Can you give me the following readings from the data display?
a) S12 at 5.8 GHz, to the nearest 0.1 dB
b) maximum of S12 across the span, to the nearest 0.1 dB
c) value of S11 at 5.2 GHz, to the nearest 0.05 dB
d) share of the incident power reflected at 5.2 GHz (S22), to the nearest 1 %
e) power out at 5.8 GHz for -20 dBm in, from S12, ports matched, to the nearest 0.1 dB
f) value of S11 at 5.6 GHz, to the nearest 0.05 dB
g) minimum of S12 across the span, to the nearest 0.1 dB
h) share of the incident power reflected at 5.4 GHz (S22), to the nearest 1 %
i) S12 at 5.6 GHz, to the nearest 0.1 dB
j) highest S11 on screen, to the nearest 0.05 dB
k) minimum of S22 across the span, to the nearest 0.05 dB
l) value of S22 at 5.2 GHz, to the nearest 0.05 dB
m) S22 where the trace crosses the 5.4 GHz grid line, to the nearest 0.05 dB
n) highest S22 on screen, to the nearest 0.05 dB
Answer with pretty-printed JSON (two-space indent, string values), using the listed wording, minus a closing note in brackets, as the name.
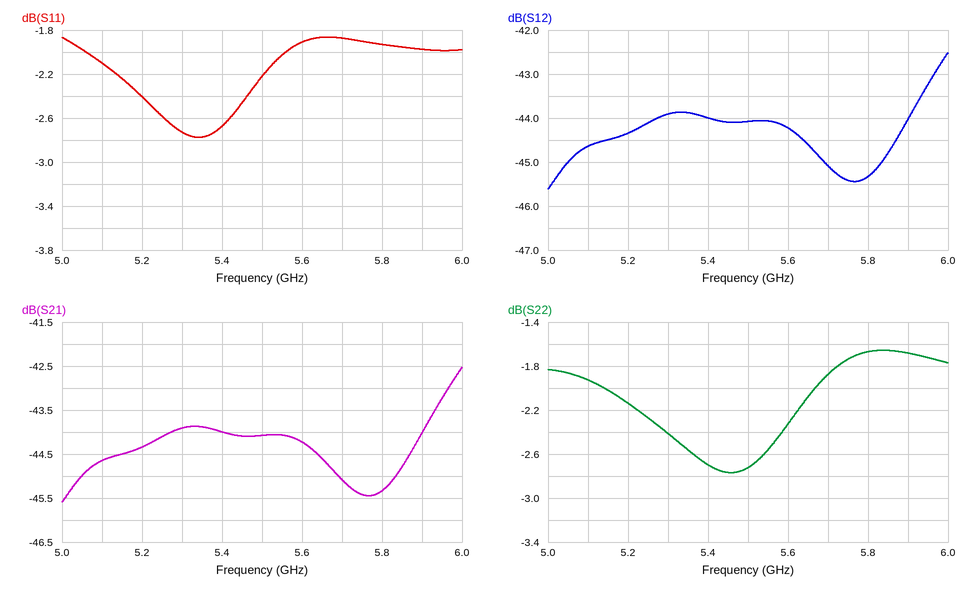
{
  "S12 at 5.8 GHz, to the nearest 0.1 dB": "-45.3 dB",
  "maximum of S12 across the span, to the nearest 0.1 dB": "-42.5 dB",
  "value of S11 at 5.2 GHz, to the nearest 0.05 dB": "-2.40 dB",
  "share of the incident power reflected at 5.2 GHz (S22), to the nearest 1 %": "61 %",
  "power out at 5.8 GHz for -20 dBm in, from S12, ports matched, to the nearest 0.1 dB": "-65.3 dBm",
  "value of S11 at 5.6 GHz, to the nearest 0.05 dB": "-1.90 dB",
  "minimum of S12 across the span, to the nearest 0.1 dB": "-45.6 dB",
  "share of the incident power reflected at 5.4 GHz (S22), to the nearest 1 %": "54 %",
  "S12 at 5.6 GHz, to the nearest 0.1 dB": "-44.2 dB",
  "highest S11 on screen, to the nearest 0.05 dB": "-1.85 dB",
  "minimum of S22 across the span, to the nearest 0.05 dB": "-2.75 dB",
  "value of S22 at 5.2 GHz, to the nearest 0.05 dB": "-2.15 dB",
  "S22 where the trace crosses the 5.4 GHz grid line, to the nearest 0.05 dB": "-2.70 dB",
  "highest S22 on screen, to the nearest 0.05 dB": "-1.65 dB"
}
